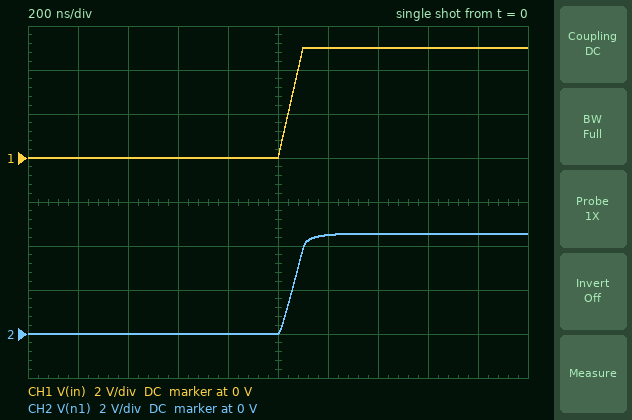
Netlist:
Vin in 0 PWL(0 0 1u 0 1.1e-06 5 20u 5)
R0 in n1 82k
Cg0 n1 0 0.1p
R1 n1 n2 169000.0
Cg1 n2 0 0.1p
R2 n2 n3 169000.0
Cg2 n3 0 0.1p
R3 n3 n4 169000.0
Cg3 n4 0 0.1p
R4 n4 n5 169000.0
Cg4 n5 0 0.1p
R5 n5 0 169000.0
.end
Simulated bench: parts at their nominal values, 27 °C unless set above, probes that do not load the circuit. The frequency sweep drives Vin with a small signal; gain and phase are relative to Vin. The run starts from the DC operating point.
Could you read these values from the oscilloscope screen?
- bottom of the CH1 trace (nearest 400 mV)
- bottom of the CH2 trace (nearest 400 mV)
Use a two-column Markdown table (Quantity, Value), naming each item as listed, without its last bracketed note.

| Quantity | Value |
|---|---|
| bottom of the CH1 trace | 0 V |
| bottom of the CH2 trace | 0 V |
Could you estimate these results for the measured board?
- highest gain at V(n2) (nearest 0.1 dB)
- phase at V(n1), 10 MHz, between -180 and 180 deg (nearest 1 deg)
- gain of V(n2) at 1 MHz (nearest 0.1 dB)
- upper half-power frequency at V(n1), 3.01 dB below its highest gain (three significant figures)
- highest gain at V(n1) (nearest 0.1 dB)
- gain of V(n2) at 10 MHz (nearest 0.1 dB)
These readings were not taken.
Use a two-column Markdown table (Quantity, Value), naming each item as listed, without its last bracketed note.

| Quantity | Value |
|---|---|
| highest gain at V(n2) | -2.7 dB |
| phase at V(n1), 10 MHz, between -180 and 180 deg | -27 deg |
| gain of V(n2) at 1 MHz | -3.1 dB |
| upper half-power frequency at V(n1), 3.01 dB below its highest gain | 12.5 MHz |
| highest gain at V(n1) | -0.8 dB |
| gain of V(n2) at 10 MHz | -9.9 dB |
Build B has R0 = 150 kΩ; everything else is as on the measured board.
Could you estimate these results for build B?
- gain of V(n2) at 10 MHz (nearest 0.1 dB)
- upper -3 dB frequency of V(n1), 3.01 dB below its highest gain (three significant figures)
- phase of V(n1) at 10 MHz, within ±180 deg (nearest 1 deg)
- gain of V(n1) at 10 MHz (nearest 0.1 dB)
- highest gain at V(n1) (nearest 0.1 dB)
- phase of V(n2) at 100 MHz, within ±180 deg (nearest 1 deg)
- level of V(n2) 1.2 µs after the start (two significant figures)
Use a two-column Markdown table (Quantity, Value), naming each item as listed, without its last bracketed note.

| Quantity | Value |
|---|---|
| gain of V(n2) at 10 MHz | -12.5 dB |
| upper -3 dB frequency of V(n1), 3.01 dB below its highest gain | 5.80 MHz |
| phase of V(n1) at 10 MHz, within ±180 deg | -38 deg |
| gain of V(n1) at 10 MHz | -5.9 dB |
| highest gain at V(n1) | -1.4 dB |
| phase of V(n2) at 100 MHz, within ±180 deg | -158 deg |
| level of V(n2) 1.2 µs after the start | 3.1 V |
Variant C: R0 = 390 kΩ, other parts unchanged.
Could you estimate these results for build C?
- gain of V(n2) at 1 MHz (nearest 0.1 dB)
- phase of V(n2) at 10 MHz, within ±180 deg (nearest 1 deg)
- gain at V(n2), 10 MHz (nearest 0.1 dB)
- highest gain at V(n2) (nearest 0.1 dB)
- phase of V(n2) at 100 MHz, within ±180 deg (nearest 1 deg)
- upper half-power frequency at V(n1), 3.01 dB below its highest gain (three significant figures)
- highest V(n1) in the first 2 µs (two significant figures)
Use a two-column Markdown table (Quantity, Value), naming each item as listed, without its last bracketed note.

| Quantity | Value |
|---|---|
| gain of V(n2) at 1 MHz | -6.3 dB |
| phase of V(n2) at 10 MHz, within ±180 deg | -92 deg |
| gain at V(n2), 10 MHz | -18.6 dB |
| highest gain at V(n2) | -5.2 dB |
| phase of V(n2) at 100 MHz, within ±180 deg | -162 deg |
| upper half-power frequency at V(n1), 3.01 dB below its highest gain | 2.39 MHz |
| highest V(n1) in the first 2 µs | 3.4 V |
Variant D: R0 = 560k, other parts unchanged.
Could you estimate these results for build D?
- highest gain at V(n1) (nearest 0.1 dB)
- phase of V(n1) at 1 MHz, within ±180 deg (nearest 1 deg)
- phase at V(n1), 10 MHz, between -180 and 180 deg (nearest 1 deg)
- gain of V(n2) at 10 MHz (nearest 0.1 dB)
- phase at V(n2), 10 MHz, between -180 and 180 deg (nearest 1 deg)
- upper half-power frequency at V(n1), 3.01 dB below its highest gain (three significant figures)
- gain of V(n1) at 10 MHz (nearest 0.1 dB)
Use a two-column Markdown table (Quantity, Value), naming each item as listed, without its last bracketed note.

| Quantity | Value |
|---|---|
| highest gain at V(n1) | -4.4 dB |
| phase of V(n1) at 1 MHz, within ±180 deg | -23 deg |
| phase at V(n1), 10 MHz, between -180 and 180 deg | -55 deg |
| gain of V(n2) at 10 MHz | -21.4 dB |
| phase at V(n2), 10 MHz, between -180 and 180 deg | -95 deg |
| upper half-power frequency at V(n1), 3.01 dB below its highest gain | 1.89 MHz |
| gain of V(n1) at 10 MHz | -14.8 dB |
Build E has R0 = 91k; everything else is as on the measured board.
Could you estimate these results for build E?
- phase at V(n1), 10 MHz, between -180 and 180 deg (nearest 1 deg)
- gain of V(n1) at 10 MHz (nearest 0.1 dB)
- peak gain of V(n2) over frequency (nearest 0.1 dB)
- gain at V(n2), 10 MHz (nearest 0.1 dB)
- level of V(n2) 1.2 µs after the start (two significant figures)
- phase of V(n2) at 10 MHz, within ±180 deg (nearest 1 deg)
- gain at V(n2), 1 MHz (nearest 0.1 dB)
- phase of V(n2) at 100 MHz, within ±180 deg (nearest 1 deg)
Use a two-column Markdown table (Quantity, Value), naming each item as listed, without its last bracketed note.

| Quantity | Value |
|---|---|
| phase at V(n1), 10 MHz, between -180 and 180 deg | -29 deg |
| gain of V(n1) at 10 MHz | -3.7 dB |
| peak gain of V(n2) over frequency | -2.8 dB |
| gain at V(n2), 10 MHz | -10.3 dB |
| level of V(n2) 1.2 µs after the start | 3.4 V |
| phase of V(n2) at 10 MHz, within ±180 deg | -68 deg |
| gain at V(n2), 1 MHz | -3.2 dB |
| phase of V(n2) at 100 MHz, within ±180 deg | -155 deg |
